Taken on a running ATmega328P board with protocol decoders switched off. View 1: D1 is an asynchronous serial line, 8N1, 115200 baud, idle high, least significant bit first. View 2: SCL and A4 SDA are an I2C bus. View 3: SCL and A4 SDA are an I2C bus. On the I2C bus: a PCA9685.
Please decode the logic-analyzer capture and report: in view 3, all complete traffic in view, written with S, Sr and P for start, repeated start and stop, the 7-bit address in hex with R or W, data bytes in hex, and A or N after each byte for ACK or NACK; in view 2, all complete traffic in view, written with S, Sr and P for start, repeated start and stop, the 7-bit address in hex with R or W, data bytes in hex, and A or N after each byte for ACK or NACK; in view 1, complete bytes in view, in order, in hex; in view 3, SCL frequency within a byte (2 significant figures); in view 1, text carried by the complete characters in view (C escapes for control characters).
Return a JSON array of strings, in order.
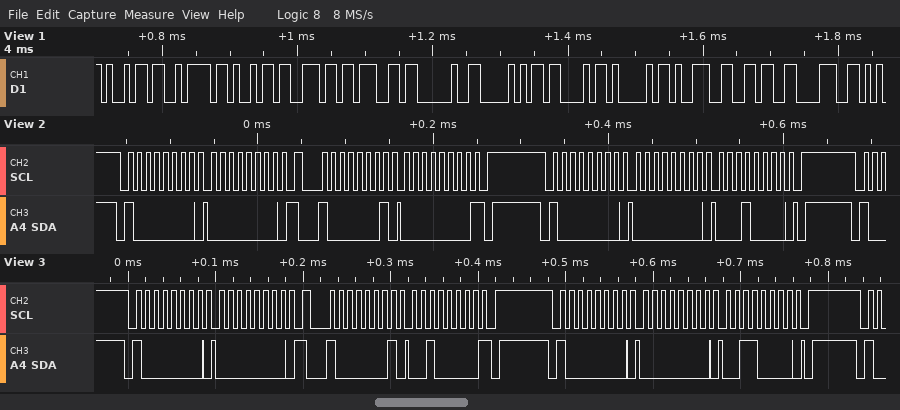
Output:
["S 40W A 00 A Sr 40R A 20 N P S 40W A 00 A 30 A P", "S 40W A 00 A Sr 40R A 00 N P S 40W A 00 A 10 A P", "69 7A 69 6E 67 20 50 43 41 39 36 38", "100 kHz", "\"izing PCA968\""]
